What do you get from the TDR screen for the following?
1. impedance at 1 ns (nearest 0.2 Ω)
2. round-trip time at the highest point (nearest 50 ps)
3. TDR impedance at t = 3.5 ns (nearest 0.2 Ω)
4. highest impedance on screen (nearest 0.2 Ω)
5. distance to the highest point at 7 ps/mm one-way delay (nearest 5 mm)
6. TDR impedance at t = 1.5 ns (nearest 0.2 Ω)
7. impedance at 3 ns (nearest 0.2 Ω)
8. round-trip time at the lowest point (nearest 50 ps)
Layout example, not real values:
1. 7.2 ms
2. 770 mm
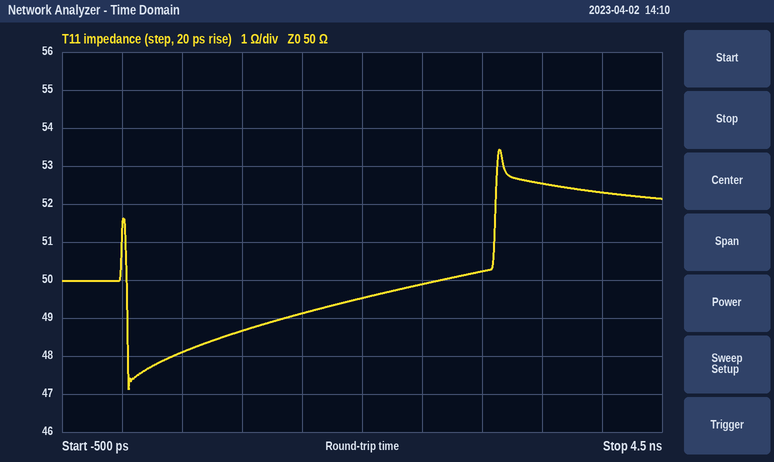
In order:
1. 48.6 Ω
2. 3.15 ns
3. 52.6 Ω
4. 53.4 Ω
5. 225 mm
6. 49.2 Ω
7. 50.2 Ω
8. 50 ps
